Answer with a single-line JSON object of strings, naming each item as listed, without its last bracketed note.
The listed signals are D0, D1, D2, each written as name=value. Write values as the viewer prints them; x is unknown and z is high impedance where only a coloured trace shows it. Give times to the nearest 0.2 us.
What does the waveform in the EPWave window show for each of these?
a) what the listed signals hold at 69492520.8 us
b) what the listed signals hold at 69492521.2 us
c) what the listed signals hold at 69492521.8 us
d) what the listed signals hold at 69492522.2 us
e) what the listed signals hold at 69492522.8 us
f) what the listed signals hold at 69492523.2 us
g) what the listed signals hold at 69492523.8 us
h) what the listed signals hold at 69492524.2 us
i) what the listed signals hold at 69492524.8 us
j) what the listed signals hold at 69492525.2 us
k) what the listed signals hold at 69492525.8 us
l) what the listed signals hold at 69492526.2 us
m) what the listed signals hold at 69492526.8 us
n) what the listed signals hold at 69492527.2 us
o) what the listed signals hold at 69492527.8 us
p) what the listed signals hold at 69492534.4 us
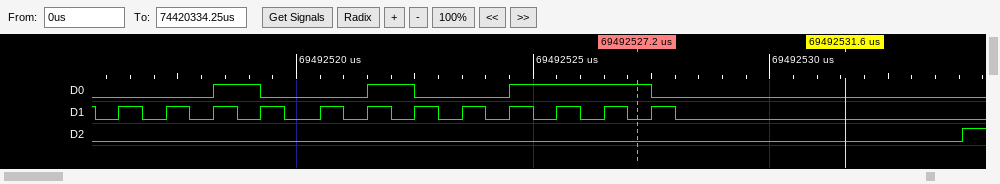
{"what the listed signals hold at 69492520.8 us": "D0=0, D1=1, D2=0", "what the listed signals hold at 69492521.2 us": "D0=0, D1=0, D2=0", "what the listed signals hold at 69492521.8 us": "D0=1, D1=1, D2=0", "what the listed signals hold at 69492522.2 us": "D0=1, D1=0, D2=0", "what the listed signals hold at 69492522.8 us": "D0=0, D1=1, D2=0", "what the listed signals hold at 69492523.2 us": "D0=0, D1=0, D2=0", "what the listed signals hold at 69492523.8 us": "D0=0, D1=1, D2=0", "what the listed signals hold at 69492524.2 us": "D0=0, D1=0, D2=0", "what the listed signals hold at 69492524.8 us": "D0=1, D1=1, D2=0", "what the listed signals hold at 69492525.2 us": "D0=1, D1=0, D2=0", "what the listed signals hold at 69492525.8 us": "D0=1, D1=1, D2=0", "what the listed signals hold at 69492526.2 us": "D0=1, D1=0, D2=0", "what the listed signals hold at 69492526.8 us": "D0=1, D1=1, D2=0", "what the listed signals hold at 69492527.2 us": "D0=1, D1=0, D2=0", "what the listed signals hold at 69492527.8 us": "D0=0, D1=1, D2=0", "what the listed signals hold at 69492534.4 us": "D0=0, D1=0, D2=1"}
